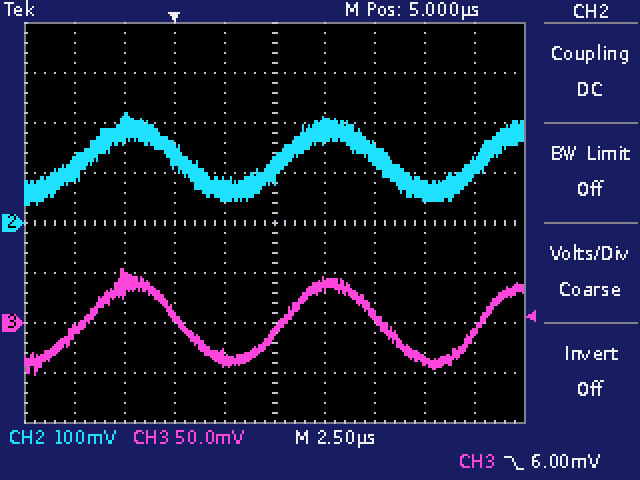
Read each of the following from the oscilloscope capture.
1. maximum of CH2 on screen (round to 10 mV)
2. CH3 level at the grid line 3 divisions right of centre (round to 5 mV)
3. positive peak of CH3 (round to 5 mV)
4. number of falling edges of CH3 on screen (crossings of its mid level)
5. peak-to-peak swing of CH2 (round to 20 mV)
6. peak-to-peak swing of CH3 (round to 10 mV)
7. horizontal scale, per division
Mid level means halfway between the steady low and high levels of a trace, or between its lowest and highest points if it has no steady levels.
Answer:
220 mV
-35 mV
55 mV
2
180 mV
110 mV
2.5 µs
